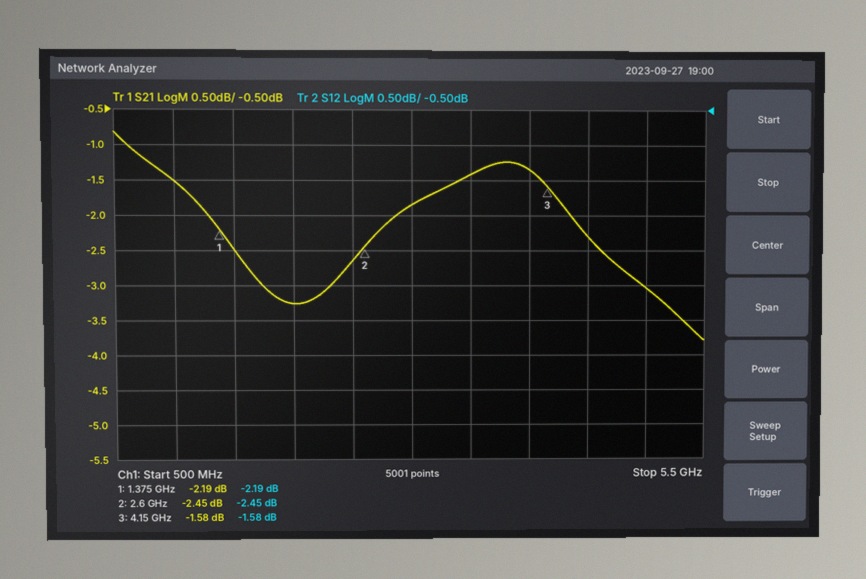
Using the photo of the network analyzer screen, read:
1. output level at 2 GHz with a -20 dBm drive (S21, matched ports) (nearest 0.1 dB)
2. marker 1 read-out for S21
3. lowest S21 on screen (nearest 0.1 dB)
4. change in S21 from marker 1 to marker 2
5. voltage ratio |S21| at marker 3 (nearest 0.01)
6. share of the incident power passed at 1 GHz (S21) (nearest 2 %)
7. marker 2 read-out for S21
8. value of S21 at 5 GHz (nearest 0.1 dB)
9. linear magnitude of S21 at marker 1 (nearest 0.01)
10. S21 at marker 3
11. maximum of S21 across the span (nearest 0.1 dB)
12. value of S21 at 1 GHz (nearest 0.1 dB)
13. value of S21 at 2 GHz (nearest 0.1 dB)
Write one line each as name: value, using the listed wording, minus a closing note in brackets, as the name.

output level at 2 GHz with a -20 dBm drive (S21, matched ports): -23.3 dBm
marker 1 read-out for S21: -2.19 dB
lowest S21 on screen: -3.8 dB
change in S21 from marker 1 to marker 2: -0.26 dB
voltage ratio |S21| at marker 3: 0.83
share of the incident power passed at 1 GHz (S21): 70 %
marker 2 read-out for S21: -2.45 dB
value of S21 at 5 GHz: -3.0 dB
linear magnitude of S21 at marker 1: 0.78
S21 at marker 3: -1.58 dB
maximum of S21 across the span: -0.8 dB
value of S21 at 1 GHz: -1.5 dB
value of S21 at 2 GHz: -3.3 dB
